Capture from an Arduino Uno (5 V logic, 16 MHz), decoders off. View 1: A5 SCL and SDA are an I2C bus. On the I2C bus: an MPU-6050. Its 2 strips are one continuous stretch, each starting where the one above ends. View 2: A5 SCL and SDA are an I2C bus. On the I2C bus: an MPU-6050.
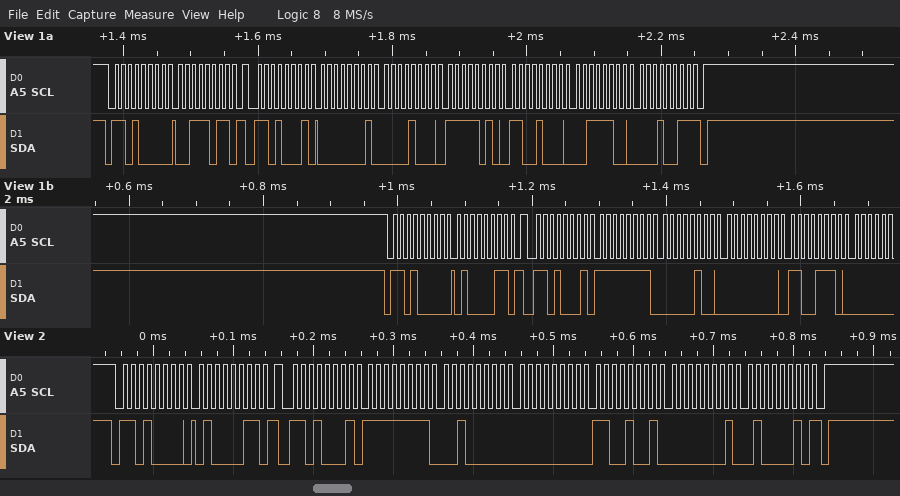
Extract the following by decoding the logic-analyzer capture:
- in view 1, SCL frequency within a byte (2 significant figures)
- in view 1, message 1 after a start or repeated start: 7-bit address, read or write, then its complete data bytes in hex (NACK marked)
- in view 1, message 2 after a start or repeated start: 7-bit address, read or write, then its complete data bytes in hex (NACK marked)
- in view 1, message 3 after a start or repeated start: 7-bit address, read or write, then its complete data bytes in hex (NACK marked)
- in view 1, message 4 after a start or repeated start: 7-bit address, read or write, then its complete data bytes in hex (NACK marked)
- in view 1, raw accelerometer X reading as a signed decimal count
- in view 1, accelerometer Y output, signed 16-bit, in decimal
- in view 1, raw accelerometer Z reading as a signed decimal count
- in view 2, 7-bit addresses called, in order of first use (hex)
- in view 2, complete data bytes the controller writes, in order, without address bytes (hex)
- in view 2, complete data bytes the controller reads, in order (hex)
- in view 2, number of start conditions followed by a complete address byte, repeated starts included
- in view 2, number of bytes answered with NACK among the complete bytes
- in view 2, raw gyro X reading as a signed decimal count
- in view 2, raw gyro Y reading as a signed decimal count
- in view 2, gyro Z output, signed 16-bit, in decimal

100 kHz
0x68 write: 3B
0x68 read: 01 08 FA C8 3C 13 NACK
0x68 write: 43
0x68 read: FF 04 00 CE
264
-1336
15379
0x68
43
FF 20 00 C9 01 42
2
1
-224
201
322
